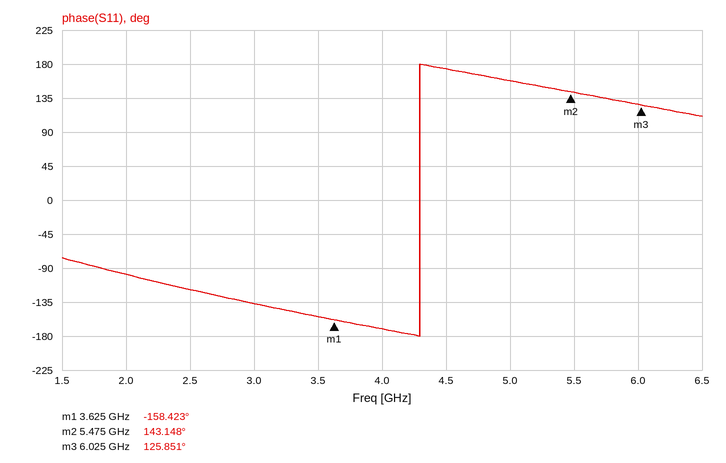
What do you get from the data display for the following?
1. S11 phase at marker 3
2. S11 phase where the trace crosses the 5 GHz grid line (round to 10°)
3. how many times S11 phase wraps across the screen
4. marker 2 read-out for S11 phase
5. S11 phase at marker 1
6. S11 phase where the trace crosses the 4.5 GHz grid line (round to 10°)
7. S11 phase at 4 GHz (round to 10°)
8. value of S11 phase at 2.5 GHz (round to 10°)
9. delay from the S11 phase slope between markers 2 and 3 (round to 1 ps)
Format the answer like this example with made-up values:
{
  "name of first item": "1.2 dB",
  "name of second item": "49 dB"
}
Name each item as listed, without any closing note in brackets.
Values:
{
  "S11 phase at marker 3": "125.851°",
  "S11 phase where the trace crosses the 5 GHz grid line": "160°",
  "how many times S11 phase wraps across the screen": "1",
  "marker 2 read-out for S11 phase": "143.148°",
  "S11 phase at marker 1": "-158.423°",
  "S11 phase where the trace crosses the 4.5 GHz grid line": "170°",
  "S11 phase at 4 GHz": "-170°",
  "value of S11 phase at 2.5 GHz": "-120°",
  "delay from the S11 phase slope between markers 2 and 3": "87 ps"
}
